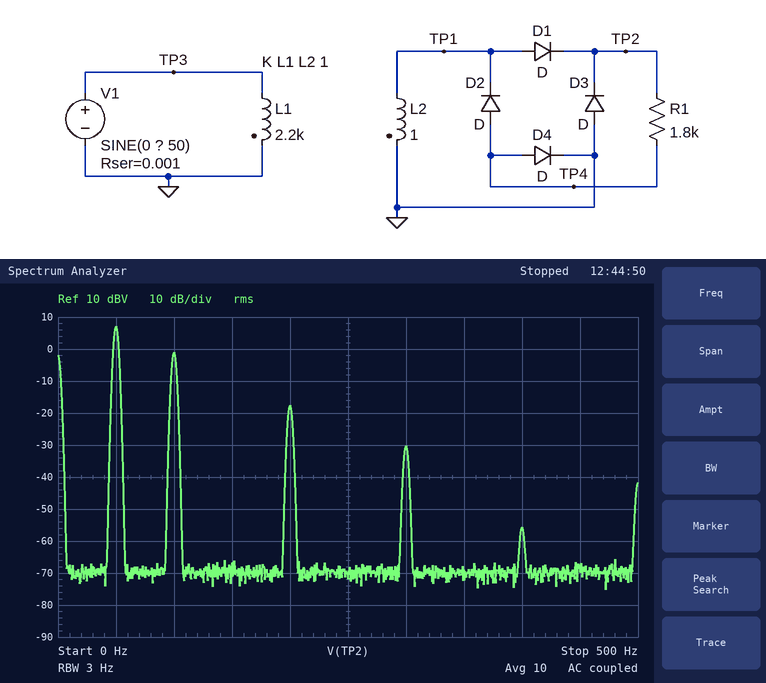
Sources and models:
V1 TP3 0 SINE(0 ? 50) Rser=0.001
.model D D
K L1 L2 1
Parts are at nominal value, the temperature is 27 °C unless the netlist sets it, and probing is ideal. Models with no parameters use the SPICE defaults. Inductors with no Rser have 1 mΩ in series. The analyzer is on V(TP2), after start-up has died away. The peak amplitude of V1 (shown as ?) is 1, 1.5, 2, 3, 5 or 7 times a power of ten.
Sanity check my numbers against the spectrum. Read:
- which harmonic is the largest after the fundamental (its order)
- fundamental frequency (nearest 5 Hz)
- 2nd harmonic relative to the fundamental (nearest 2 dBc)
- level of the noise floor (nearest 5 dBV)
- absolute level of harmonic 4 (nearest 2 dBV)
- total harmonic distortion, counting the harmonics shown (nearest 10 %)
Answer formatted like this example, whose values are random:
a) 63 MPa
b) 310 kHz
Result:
a) 2
b) 50 Hz
c) -8 dBc
d) -70 dBV
e) -18 dBV
f) 40 %
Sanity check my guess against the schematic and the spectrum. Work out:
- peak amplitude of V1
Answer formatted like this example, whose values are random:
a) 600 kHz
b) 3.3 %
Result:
a) 300 V
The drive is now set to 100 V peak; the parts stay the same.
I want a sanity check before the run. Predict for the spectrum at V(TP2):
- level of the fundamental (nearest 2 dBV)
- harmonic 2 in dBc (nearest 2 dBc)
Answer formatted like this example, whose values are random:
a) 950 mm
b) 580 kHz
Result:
a) -2 dBV
b) -14 dBc
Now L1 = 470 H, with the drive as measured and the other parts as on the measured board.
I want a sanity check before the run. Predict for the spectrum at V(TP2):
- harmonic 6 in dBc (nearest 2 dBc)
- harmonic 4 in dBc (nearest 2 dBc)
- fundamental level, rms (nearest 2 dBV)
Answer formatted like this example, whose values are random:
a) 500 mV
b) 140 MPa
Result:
a) -30 dBc
b) -22 dBc
c) 14 dBV
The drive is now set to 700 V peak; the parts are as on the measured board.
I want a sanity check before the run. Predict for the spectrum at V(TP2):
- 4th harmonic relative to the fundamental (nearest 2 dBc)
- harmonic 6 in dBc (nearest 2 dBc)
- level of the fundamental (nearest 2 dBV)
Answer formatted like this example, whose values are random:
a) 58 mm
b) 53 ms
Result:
a) -22 dBc
b) -30 dBc
c) 14 dBV
